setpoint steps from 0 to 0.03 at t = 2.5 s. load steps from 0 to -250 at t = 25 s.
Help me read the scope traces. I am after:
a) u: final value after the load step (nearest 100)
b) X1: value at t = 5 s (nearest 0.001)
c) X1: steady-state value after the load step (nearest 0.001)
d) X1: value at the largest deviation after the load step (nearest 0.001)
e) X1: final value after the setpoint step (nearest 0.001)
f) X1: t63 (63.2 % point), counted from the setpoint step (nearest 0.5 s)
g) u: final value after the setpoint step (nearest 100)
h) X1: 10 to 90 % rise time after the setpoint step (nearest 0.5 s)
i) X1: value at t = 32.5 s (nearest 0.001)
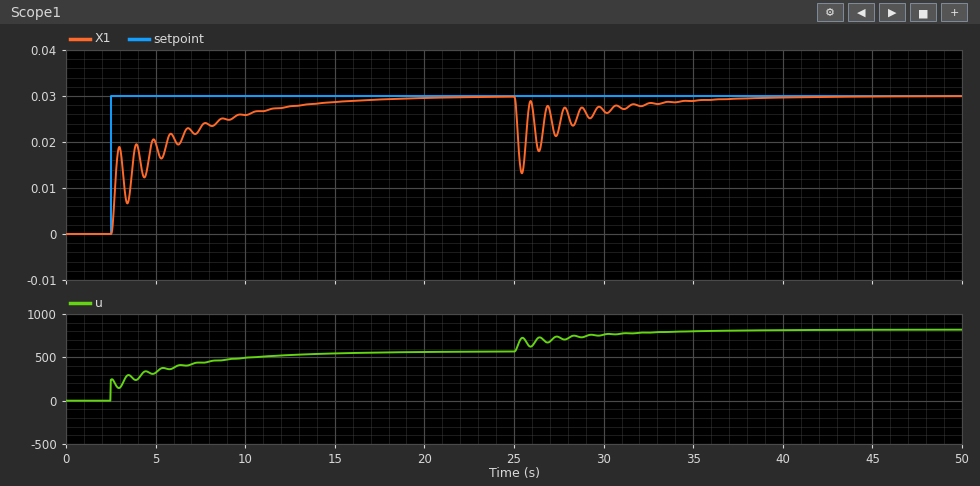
800
0.020
0.030
0.013
0.030
1.5 s
600
8.5 s
0.028
